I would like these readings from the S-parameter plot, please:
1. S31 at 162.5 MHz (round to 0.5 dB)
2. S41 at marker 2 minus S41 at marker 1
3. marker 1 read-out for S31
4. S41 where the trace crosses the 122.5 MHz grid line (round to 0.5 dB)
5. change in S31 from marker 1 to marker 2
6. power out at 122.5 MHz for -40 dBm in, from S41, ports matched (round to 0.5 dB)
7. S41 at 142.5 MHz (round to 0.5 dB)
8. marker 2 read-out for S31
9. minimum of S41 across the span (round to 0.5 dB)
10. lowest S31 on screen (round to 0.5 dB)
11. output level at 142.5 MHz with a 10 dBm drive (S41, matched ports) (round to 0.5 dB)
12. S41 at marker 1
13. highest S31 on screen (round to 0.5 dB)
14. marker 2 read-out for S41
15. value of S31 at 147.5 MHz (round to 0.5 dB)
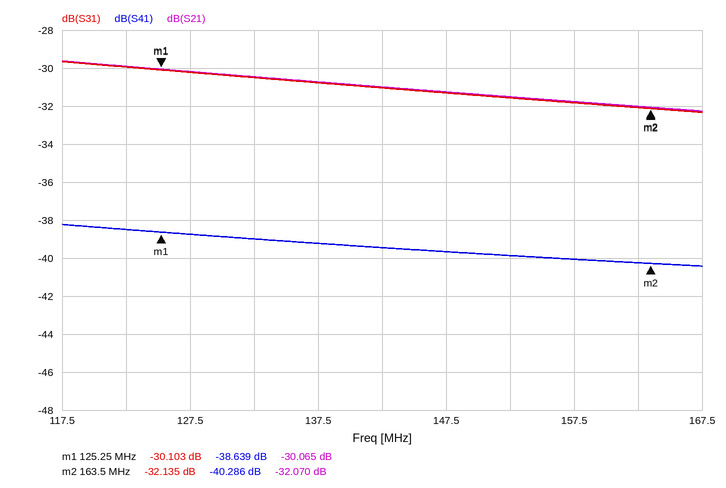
-32.0 dB
-1.647 dB
-30.103 dB
-38.5 dB
-2.032 dB
-78.5 dBm
-39.5 dB
-32.135 dB
-40.5 dB
-32.5 dB
-29.5 dBm
-38.639 dB
-29.5 dB
-40.286 dB
-31.5 dB
